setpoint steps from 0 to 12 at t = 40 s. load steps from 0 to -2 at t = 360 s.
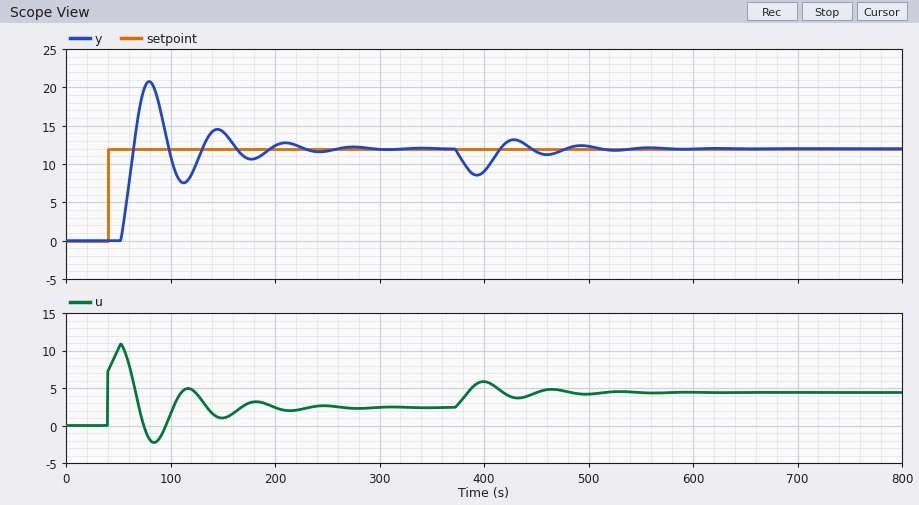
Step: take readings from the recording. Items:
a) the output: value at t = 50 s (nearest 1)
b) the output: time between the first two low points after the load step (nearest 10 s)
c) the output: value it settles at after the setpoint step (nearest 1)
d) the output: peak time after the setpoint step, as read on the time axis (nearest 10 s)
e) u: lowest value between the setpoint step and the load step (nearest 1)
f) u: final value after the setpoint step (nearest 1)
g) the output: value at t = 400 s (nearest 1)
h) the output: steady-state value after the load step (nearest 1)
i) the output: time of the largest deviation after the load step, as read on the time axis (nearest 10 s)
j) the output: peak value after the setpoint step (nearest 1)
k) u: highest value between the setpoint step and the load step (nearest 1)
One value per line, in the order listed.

0
70 s
12
80 s
-2
2
9
12
390 s
21
11
